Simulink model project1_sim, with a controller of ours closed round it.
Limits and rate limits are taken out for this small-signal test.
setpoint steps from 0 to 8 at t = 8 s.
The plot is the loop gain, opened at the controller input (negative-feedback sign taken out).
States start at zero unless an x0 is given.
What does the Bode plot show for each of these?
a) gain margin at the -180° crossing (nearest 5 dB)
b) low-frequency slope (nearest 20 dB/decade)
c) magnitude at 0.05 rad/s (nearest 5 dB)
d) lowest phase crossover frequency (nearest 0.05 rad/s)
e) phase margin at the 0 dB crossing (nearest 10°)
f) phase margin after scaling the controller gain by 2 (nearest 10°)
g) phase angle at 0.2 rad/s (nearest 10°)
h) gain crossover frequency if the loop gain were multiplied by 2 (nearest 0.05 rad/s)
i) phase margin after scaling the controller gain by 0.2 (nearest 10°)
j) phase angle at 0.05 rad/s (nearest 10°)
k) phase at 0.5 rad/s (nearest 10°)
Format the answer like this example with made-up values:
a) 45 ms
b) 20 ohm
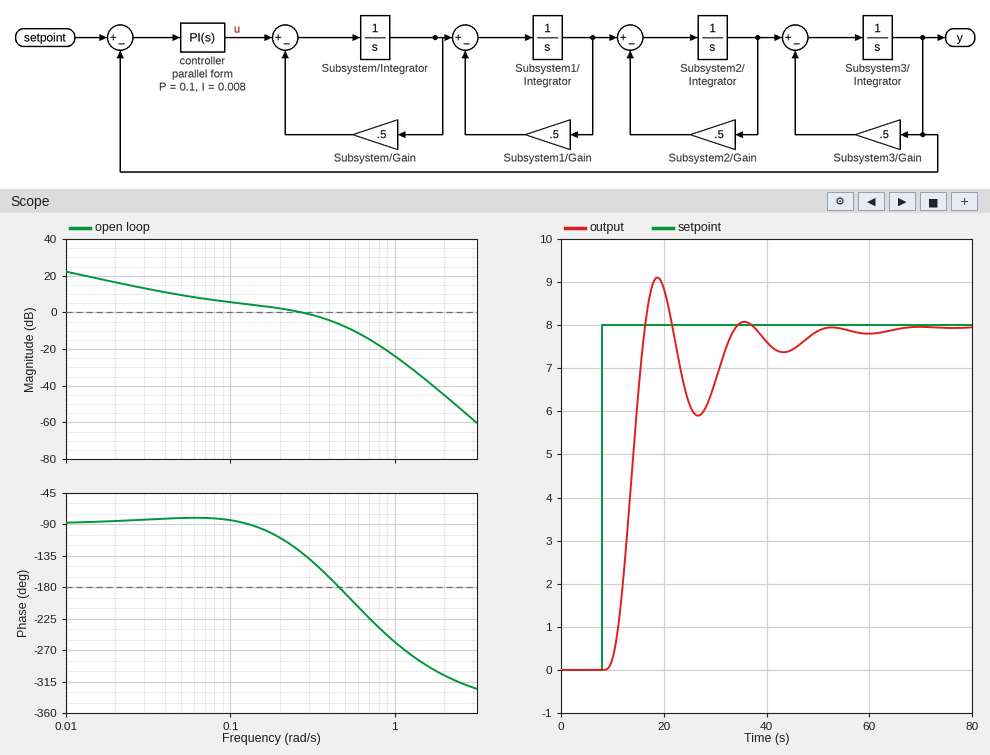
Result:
a) 5 dB
b) -20 dB/decade
c) 10 dB
d) 0.45 rad/s
e) 50°
f) 0°
g) -110°
h) 0.45 rad/s
i) 100°
j) -80°
k) -190°
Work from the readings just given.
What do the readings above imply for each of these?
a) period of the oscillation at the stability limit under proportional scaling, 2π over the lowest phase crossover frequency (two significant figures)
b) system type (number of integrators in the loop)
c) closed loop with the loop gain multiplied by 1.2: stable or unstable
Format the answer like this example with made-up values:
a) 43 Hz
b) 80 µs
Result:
a) 14 s
b) 1
c) stable
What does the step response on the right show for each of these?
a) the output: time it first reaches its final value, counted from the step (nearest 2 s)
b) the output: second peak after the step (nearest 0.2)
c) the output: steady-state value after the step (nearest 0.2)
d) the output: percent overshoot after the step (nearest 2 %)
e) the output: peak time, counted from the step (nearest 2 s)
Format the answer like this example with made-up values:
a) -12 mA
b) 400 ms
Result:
a) 8 s
b) 8.0
c) 8.0
d) 14 %
e) 10 s
